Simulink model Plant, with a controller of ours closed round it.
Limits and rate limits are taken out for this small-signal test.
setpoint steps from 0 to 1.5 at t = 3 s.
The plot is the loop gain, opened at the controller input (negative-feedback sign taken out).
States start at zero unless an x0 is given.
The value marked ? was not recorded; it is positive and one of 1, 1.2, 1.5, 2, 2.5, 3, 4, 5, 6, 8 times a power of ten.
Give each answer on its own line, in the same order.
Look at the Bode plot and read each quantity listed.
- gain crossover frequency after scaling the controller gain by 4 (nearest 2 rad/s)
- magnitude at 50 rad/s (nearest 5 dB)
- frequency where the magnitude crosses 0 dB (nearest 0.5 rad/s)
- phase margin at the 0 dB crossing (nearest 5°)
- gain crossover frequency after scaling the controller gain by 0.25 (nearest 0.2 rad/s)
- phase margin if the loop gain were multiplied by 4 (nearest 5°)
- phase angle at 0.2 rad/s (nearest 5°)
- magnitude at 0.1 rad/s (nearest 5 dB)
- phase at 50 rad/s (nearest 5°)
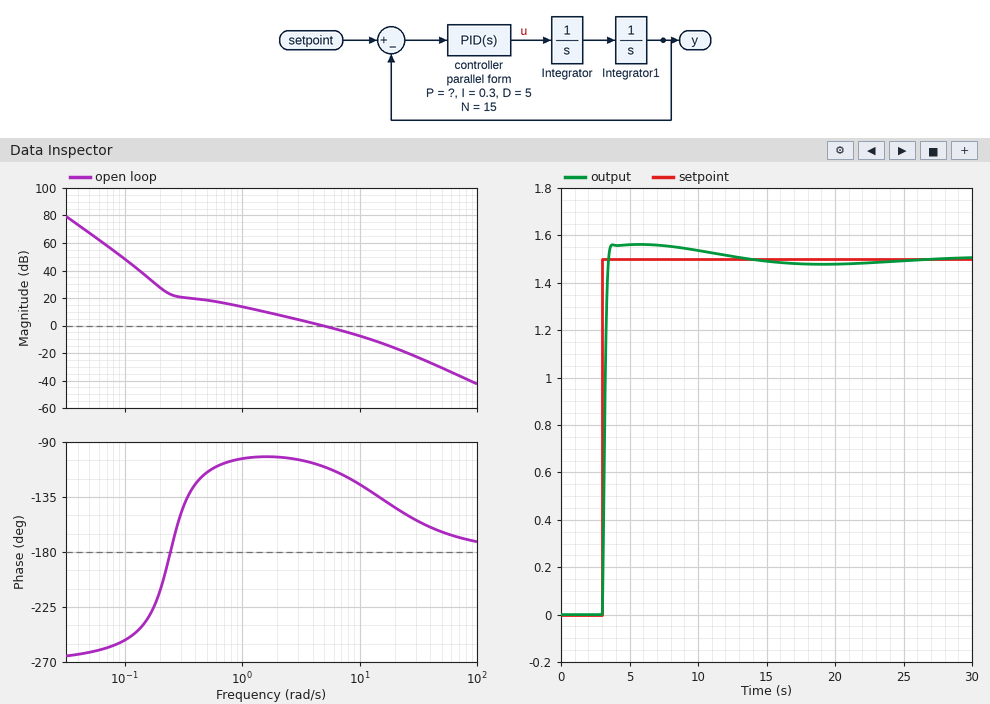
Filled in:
14 rad/s
-30 dB
5.0 rad/s
70°
1.2 rad/s
45°
-210°
50 dB
-165°
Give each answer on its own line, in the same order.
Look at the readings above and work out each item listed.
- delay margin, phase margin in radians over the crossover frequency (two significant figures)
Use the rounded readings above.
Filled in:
0.24 s
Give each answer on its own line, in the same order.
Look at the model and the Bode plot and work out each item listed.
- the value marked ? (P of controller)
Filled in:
0.8
